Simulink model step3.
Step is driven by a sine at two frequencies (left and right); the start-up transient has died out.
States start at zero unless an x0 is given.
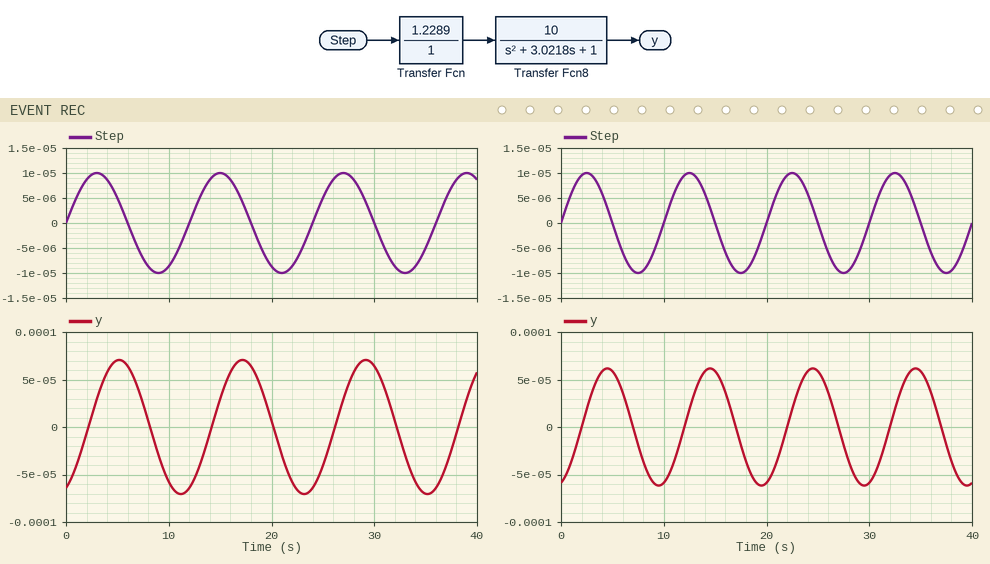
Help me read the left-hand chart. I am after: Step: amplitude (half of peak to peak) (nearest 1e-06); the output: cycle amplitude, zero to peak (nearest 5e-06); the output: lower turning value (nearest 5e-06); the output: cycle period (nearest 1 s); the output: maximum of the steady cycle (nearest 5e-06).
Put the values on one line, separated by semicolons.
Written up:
0.000010; 0.000070; -0.000070; 12 s; 0.000070
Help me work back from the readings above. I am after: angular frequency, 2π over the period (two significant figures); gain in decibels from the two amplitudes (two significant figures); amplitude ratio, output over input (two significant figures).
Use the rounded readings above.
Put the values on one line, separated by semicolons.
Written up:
0.52 rad/s; 17 dB; 7.0
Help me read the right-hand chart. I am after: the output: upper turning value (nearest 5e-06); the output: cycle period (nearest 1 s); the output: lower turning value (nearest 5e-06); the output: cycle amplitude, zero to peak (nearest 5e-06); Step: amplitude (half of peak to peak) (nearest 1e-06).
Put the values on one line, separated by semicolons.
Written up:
0.000060; 10 s; -0.000060; 0.000060; 0.000010
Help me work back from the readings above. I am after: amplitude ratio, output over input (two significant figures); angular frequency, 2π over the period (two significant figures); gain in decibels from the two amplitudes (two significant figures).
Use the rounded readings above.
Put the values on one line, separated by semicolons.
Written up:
6.0; 0.63 rad/s; 16 dB
